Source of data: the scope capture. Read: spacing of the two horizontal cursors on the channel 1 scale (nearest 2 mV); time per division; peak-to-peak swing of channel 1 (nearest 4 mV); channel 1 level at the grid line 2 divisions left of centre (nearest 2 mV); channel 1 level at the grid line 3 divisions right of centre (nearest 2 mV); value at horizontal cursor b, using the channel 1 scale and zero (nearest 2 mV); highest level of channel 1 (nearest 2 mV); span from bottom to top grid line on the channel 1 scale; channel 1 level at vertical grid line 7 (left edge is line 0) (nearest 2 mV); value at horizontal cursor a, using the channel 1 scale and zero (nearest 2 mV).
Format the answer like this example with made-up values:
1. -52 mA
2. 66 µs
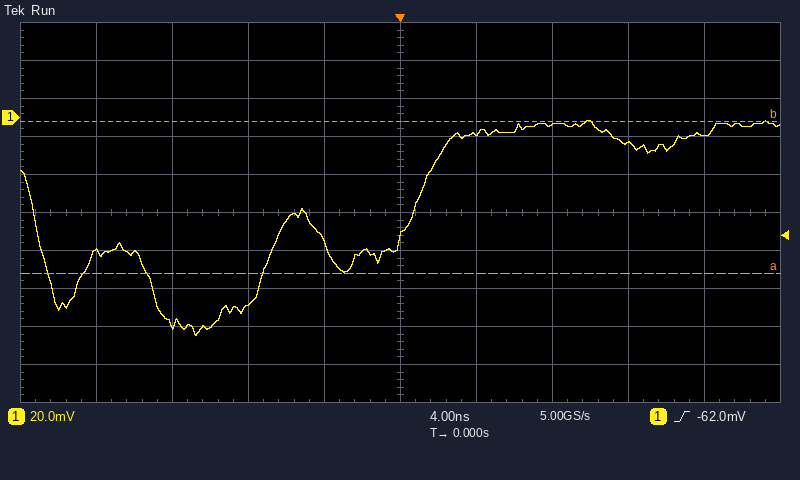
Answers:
1. 80 mV
2. 4 ns
3. 112 mV
4. -98 mV
5. -14 mV
6. -2 mV
7. -2 mV
8. 200 mV
9. -4 mV
10. -82 mV
